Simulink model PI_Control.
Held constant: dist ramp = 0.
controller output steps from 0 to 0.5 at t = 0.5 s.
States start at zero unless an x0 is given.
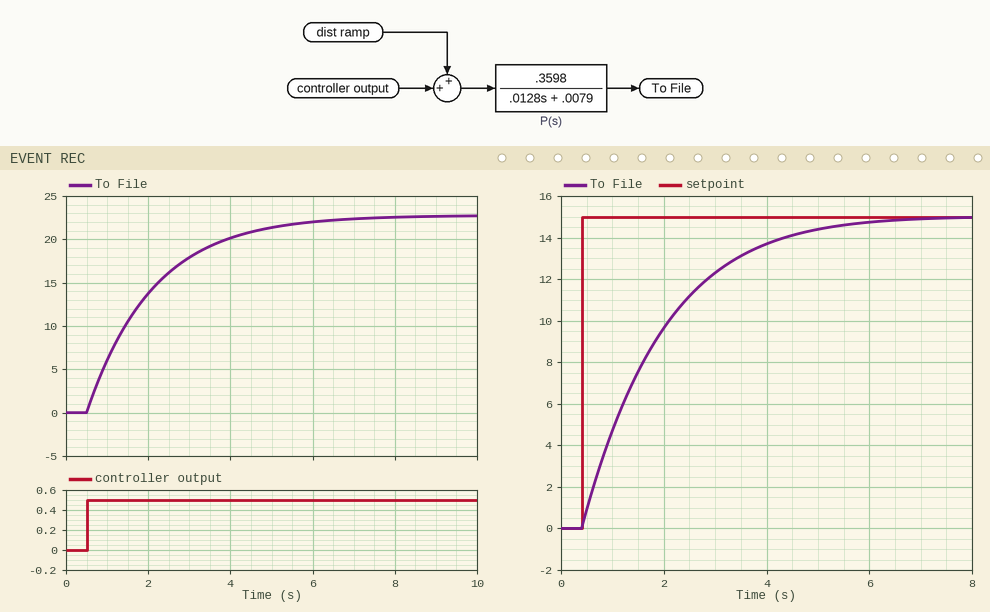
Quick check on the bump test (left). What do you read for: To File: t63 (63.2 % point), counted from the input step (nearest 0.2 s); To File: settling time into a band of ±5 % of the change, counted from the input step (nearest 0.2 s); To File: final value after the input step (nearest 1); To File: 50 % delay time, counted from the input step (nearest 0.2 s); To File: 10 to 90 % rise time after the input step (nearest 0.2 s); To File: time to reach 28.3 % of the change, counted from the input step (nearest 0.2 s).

1.6 s
4.8 s
23
1.2 s
3.6 s
0.6 s
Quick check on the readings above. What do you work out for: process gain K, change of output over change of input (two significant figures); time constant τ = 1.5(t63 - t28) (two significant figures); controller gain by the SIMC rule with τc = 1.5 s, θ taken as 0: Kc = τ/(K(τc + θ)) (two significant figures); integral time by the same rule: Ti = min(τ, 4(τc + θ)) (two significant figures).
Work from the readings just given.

46
1.5 s
0.022
1.5 s
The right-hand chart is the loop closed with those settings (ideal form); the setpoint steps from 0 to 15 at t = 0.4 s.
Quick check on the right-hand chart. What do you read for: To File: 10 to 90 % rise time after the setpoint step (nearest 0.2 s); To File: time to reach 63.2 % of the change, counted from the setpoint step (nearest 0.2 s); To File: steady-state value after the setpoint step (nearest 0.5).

3.2 s
1.6 s
15.0
